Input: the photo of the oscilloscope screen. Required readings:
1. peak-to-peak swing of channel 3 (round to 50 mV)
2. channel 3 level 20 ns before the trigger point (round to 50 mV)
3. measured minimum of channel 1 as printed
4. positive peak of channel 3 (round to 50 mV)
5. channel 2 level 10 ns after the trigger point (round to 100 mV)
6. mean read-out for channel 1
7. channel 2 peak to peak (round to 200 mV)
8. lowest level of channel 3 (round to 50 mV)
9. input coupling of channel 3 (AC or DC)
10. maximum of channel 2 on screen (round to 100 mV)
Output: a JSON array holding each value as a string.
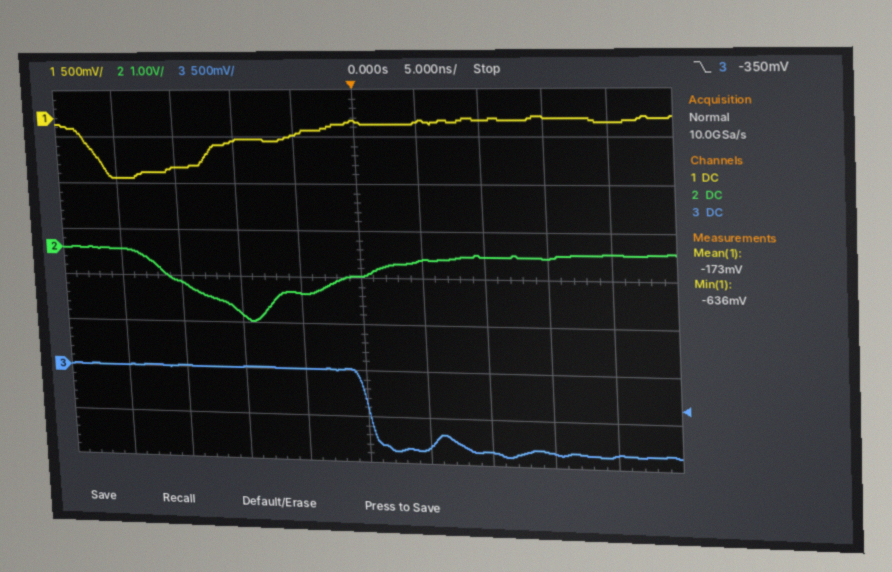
["900 mV", "0 mV", "-636 mV", "0 mV", "-100 mV", "-173 mV", "1.6 V", "-900 mV", "DC", "0.0 V"]
